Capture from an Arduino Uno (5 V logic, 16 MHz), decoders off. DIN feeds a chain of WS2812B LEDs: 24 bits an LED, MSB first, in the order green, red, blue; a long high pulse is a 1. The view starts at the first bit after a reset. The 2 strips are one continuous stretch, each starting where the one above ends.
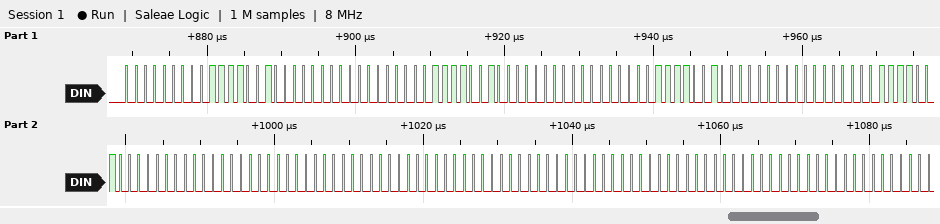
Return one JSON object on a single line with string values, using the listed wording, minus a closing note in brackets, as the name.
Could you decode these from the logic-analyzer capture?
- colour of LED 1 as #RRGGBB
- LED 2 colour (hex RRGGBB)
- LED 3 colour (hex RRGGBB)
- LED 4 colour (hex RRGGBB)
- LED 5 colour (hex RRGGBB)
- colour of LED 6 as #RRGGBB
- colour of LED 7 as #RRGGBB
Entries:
{"colour of LED 1 as #RRGGBB": "#790000", "LED 2 colour": "#790000", "LED 3 colour": "#790000", "LED 4 colour": "#790000", "LED 5 colour": "#000000", "colour of LED 6 as #RRGGBB": "#000000", "colour of LED 7 as #RRGGBB": "#000000"}
